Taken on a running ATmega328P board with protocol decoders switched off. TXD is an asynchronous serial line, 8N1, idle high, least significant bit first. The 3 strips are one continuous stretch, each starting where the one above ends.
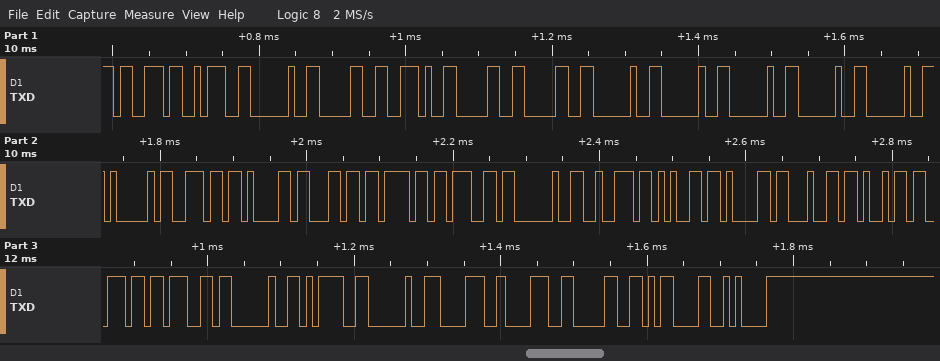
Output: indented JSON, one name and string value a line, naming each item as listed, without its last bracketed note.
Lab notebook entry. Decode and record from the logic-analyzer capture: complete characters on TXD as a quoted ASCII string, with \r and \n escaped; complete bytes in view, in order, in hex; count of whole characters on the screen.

{
  "complete characters on TXD as a quoted ASCII string, with \\r and \\n escaped": "\"s: 0.00     Analog reading = 880\\r\\n\"",
  "complete bytes in view, in order, in hex": "73 3A 20 30 2E 30 30 20 20 20 20 20 41 6E 61 6C 6F 67 20 72 65 61 64 69 6E 67 20 3D 20 38 38 30 0D 0A",
  "count of whole characters on the screen": "34"
}
